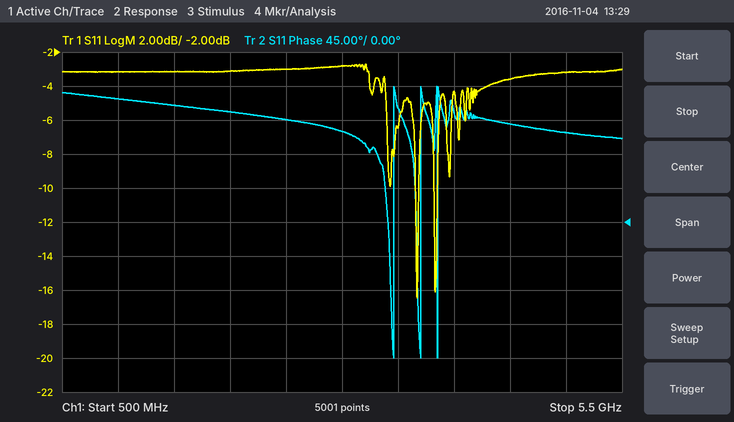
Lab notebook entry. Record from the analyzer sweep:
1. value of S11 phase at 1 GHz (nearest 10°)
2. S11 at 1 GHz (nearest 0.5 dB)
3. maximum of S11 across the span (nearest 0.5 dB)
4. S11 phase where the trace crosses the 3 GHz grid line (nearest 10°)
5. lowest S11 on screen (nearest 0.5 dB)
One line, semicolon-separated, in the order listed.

160°; -3.0 dB; -2.5 dB; 120°; -16.5 dB
